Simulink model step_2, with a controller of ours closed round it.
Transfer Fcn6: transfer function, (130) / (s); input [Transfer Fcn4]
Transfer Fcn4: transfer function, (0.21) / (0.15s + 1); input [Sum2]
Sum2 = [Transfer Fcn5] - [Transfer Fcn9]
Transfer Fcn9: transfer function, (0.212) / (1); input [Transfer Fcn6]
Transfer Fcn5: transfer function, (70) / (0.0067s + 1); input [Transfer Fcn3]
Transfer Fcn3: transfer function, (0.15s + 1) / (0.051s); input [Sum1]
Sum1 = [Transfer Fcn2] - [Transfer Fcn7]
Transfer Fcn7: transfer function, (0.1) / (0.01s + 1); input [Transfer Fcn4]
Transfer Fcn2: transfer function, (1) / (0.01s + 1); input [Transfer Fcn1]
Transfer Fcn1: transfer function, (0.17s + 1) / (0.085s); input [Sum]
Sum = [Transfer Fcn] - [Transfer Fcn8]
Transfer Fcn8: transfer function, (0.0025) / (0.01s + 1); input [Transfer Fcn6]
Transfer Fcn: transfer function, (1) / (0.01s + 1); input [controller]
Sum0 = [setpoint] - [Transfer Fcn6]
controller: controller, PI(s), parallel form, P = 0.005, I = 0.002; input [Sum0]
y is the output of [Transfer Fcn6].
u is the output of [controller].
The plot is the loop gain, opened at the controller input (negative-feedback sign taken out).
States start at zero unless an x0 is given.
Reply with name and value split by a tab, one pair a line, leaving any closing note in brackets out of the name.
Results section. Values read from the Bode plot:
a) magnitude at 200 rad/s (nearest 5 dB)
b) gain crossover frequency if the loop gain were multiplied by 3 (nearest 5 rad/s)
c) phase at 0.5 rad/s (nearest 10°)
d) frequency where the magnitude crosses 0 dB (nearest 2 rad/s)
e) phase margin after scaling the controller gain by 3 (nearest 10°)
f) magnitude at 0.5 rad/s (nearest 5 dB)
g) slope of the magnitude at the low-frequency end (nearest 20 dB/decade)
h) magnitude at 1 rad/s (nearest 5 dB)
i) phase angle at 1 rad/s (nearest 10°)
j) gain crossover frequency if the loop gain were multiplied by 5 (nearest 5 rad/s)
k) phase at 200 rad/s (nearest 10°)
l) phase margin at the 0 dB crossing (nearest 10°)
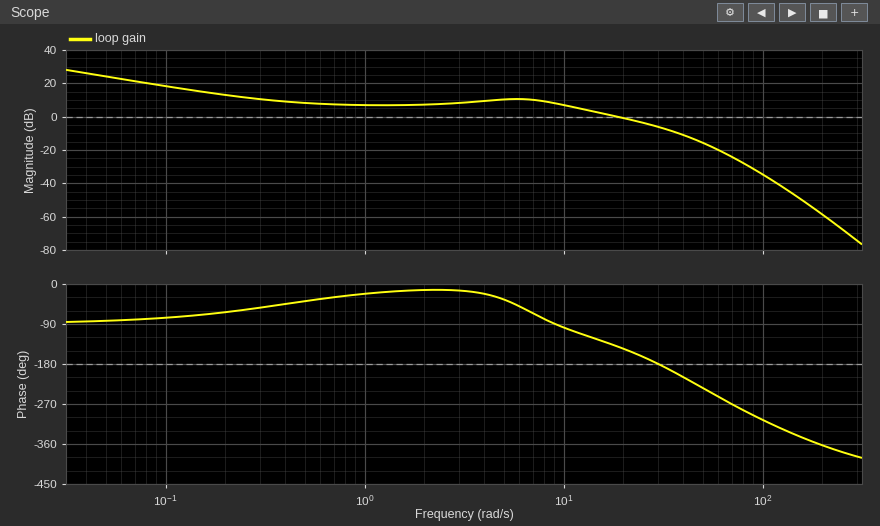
magnitude at 200 rad/s	-60 dB
gain crossover frequency if the loop gain were multiplied by 3	35 rad/s
phase at 0.5 rad/s	-40°
frequency where the magnitude crosses 0 dB	18 rad/s
phase margin after scaling the controller gain by 3	-20°
magnitude at 0.5 rad/s	10 dB
slope of the magnitude at the low-frequency end	-20 dB/decade
magnitude at 1 rad/s	5 dB
phase angle at 1 rad/s	-20°
gain crossover frequency if the loop gain were multiplied by 5	45 rad/s
phase at 200 rad/s	-360°
phase margin at the 0 dB crossing	40°
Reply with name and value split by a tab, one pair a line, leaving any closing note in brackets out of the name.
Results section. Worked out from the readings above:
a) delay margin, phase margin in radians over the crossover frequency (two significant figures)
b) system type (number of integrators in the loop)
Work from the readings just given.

delay margin, phase margin in radians over the crossover frequency	0.039 s
system type	1
